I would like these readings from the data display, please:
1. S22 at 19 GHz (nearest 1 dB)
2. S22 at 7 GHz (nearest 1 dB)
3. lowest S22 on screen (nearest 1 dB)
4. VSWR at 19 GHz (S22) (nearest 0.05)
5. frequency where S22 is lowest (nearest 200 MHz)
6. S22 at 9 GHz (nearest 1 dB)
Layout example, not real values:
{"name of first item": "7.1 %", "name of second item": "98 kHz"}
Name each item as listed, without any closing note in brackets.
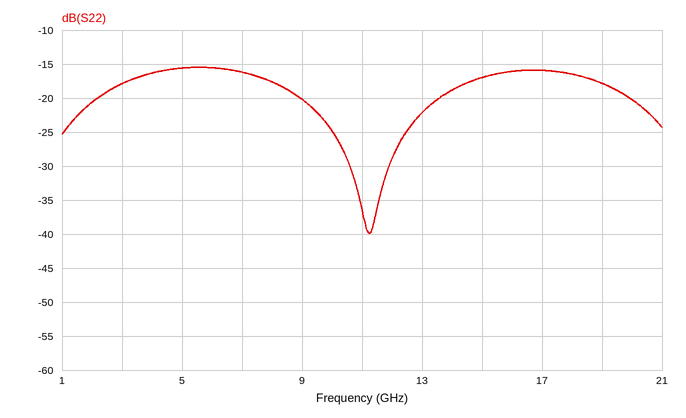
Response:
{"S22 at 19 GHz": "-18 dB", "S22 at 7 GHz": "-16 dB", "lowest S22 on screen": "-40 dB", "VSWR at 19 GHz (S22)": "1.30", "frequency where S22 is lowest": "11.2 GHz", "S22 at 9 GHz": "-20 dB"}
